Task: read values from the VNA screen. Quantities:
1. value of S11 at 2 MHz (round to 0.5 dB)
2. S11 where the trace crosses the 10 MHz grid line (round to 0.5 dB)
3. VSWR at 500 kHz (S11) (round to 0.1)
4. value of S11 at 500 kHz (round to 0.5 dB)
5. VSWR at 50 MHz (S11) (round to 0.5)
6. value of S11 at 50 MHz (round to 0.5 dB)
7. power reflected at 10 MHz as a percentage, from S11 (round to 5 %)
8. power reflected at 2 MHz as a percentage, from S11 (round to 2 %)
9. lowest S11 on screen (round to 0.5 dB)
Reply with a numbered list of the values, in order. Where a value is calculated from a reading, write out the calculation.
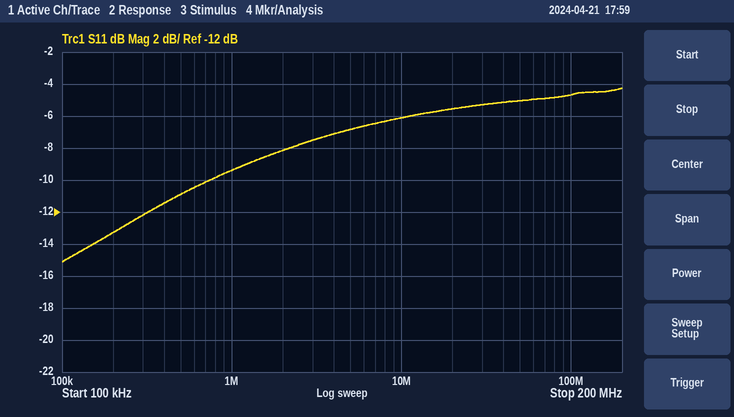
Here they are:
1. -8.0 dB
2. -6.0 dB
3. |Γ| = 10^(-11/20) = 0.2818; VSWR = (1 + 0.2818)/(1 − 0.2818) ≈ 1.8
4. -11.0 dB
5. |Γ| = 10^(-5/20) = 0.5623; VSWR = (1 + 0.5623)/(1 − 0.5623) ≈ 3.57, so 3.5 to the nearest 0.5
6. -5.0 dB
7. 10^(-6/10) ≈ 25 %
8. 10^(-8/10) ≈ 16 %
9. -15.0 dB
